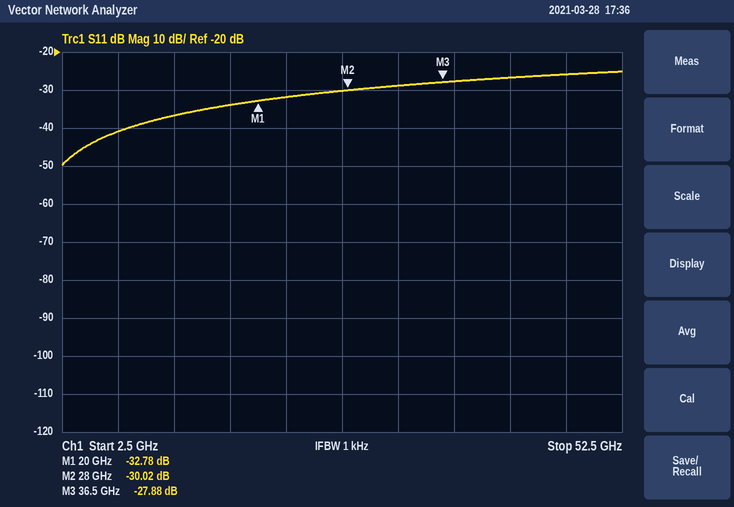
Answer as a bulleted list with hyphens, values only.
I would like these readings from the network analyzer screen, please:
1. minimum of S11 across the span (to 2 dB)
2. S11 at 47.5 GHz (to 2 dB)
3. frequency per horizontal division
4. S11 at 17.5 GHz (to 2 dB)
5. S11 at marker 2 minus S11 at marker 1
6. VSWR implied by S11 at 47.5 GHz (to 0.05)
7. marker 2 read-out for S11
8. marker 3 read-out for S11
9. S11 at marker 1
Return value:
- -50 dB
- -26 dB
- 5 GHz
- -34 dB
- 2.76 dB
- 1.10
- -30.02 dB
- -27.88 dB
- -32.78 dB
